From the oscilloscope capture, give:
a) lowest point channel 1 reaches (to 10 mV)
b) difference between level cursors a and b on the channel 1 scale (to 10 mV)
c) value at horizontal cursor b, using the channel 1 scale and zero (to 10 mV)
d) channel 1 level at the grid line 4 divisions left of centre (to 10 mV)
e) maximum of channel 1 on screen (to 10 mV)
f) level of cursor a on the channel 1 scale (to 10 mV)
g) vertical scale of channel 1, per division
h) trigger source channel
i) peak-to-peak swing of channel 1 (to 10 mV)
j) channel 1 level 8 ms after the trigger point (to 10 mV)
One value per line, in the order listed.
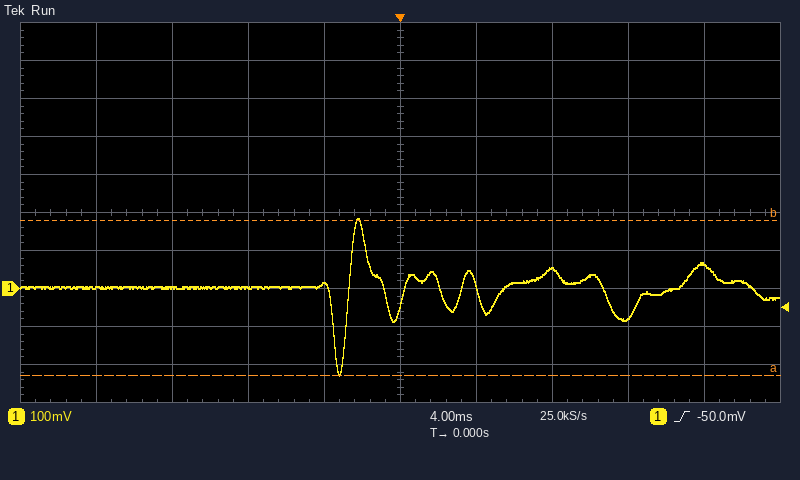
-230 mV
410 mV
180 mV
0 mV
180 mV
-230 mV
100 mV
channel 1
410 mV
50 mV
